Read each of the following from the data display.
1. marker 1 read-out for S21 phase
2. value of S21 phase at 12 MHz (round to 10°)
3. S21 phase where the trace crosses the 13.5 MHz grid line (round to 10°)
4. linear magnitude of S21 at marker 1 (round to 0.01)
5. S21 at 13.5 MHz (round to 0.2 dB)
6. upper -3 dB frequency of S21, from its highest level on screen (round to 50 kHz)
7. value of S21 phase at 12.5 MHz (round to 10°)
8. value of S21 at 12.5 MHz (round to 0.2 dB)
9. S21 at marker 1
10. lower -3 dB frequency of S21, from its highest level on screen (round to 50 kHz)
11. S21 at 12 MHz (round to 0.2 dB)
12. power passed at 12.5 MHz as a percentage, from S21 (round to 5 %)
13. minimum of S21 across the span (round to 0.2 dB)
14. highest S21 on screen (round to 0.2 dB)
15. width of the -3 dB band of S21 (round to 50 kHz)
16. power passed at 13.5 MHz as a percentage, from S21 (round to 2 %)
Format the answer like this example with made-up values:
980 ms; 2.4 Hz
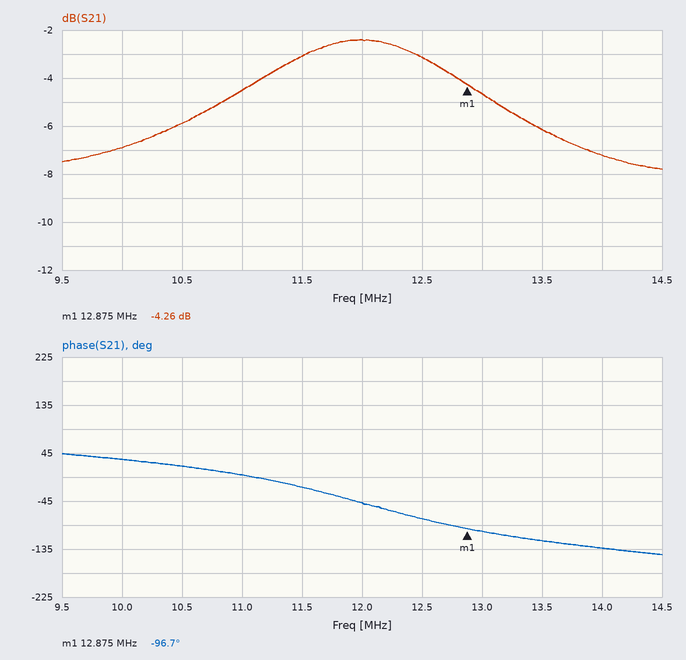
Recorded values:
-96.7°; -50°; -120°; 0.61; -6.2 dB; 13.25 MHz; -80°; -3.2 dB; -4.26 dB; 10.70 MHz; -2.4 dB; 50 %; -7.8 dB; -2.4 dB; 2.55 MHz; 24 %
